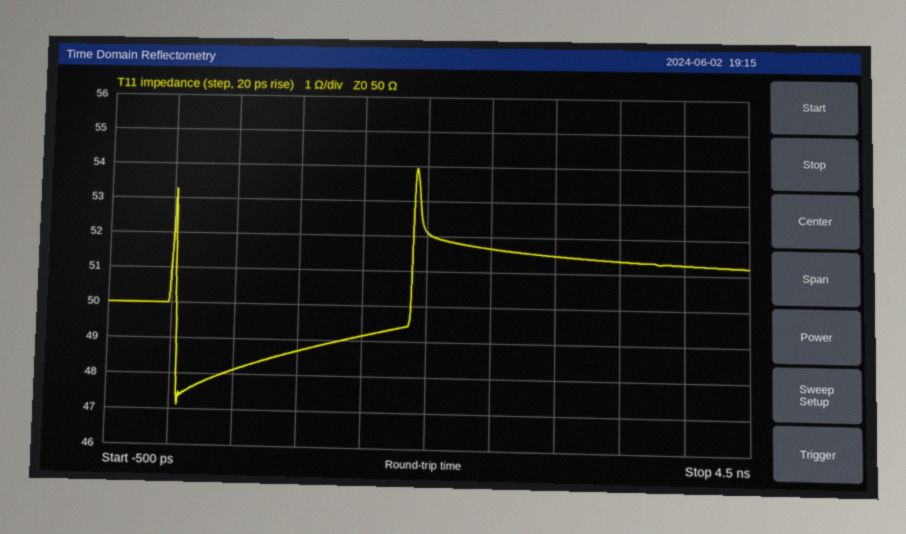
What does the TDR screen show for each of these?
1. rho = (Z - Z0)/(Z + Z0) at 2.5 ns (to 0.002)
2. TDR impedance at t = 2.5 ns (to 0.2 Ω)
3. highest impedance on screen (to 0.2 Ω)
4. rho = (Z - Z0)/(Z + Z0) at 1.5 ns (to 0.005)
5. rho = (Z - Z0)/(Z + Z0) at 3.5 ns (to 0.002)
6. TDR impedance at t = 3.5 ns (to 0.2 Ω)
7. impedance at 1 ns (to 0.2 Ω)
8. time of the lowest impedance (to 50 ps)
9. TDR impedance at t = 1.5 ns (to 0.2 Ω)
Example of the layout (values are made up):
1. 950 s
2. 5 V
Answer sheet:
1. +0.016
2. 51.6 Ω
3. 54.0 Ω
4. -0.010
5. +0.014
6. 51.4 Ω
7. 48.6 Ω
8. 50 ps
9. 49.2 Ω
